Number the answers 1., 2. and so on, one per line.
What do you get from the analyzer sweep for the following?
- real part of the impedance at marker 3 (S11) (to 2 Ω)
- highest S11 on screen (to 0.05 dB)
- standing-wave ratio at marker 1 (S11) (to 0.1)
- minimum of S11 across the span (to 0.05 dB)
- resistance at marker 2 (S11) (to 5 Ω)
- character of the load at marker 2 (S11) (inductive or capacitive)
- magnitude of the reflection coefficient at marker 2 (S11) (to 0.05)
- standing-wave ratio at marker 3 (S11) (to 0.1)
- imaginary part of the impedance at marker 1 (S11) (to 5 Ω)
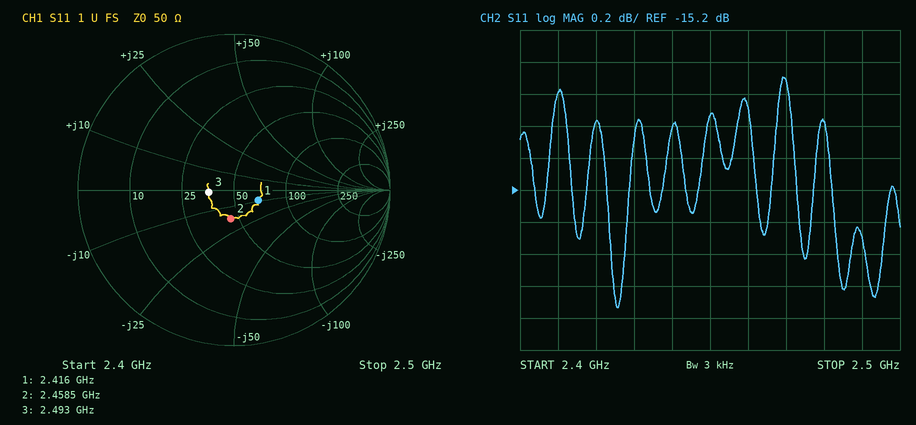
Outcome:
1. 36 Ω
2. -14.50 dB
3. 1.4
4. -15.95 dB
5. 45 Ω
6. capacitive
7. 0.20
8. 1.4
9. -10 Ω
